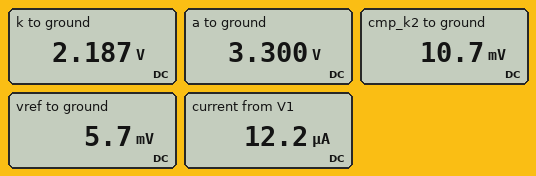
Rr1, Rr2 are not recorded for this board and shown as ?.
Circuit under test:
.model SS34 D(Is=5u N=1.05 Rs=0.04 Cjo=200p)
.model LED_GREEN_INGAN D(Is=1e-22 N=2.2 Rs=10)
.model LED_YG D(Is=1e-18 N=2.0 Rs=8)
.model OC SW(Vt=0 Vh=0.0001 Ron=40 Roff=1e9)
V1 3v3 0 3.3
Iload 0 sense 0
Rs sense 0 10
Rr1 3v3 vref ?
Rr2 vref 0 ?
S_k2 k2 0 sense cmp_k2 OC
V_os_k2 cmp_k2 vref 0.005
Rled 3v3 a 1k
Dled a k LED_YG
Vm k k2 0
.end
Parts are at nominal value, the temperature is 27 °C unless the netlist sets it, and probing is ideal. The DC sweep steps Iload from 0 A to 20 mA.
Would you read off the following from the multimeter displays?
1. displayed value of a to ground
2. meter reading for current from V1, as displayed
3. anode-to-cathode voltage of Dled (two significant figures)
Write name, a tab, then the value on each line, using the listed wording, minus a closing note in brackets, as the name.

displayed value of a to ground	3.300 V
meter reading for current from V1, as displayed	12.2 µA
anode-to-cathode voltage of Dled	1.1 V
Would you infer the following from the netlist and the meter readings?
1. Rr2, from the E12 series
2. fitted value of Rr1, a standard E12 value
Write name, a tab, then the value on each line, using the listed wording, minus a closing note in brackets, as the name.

Rr2, from the E12 series	470 Ω
fitted value of Rr1, a standard E12 value	270 kΩ
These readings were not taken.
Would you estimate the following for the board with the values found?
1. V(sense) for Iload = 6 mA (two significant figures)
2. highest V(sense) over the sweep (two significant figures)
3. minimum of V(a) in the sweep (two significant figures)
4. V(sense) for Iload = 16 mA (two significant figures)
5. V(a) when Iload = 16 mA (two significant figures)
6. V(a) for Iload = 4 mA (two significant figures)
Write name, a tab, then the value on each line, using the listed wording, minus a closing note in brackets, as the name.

V(sense) for Iload = 6 mA	60 mV
highest V(sense) over the sweep	200 mV
minimum of V(a) in the sweep	1.9 V
V(sense) for Iload = 16 mA	160 mV
V(a) when Iload = 16 mA	1.9 V
V(a) for Iload = 4 mA	1.9 V
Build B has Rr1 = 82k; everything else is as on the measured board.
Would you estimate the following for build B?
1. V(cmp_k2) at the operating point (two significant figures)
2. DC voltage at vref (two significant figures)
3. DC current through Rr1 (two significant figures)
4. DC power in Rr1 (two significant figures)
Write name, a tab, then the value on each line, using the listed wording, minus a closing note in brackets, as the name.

V(cmp_k2) at the operating point	24 mV
DC voltage at vref	19 mV
DC current through Rr1	40 µA
DC power in Rr1	130 µW
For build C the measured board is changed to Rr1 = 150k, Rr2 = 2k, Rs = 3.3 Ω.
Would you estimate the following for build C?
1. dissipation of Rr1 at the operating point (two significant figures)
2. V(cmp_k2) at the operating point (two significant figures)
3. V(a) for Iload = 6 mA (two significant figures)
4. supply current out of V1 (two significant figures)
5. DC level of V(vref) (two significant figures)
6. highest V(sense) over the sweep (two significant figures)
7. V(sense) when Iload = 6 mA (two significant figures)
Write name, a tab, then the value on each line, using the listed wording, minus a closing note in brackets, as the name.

dissipation of Rr1 at the operating point	71 µW
V(cmp_k2) at the operating point	48 mV
V(a) for Iload = 6 mA	3.3 V
supply current out of V1	22 µA
DC level of V(vref)	43 mV
highest V(sense) over the sweep	66 mV
V(sense) when Iload = 6 mA	20 mV
